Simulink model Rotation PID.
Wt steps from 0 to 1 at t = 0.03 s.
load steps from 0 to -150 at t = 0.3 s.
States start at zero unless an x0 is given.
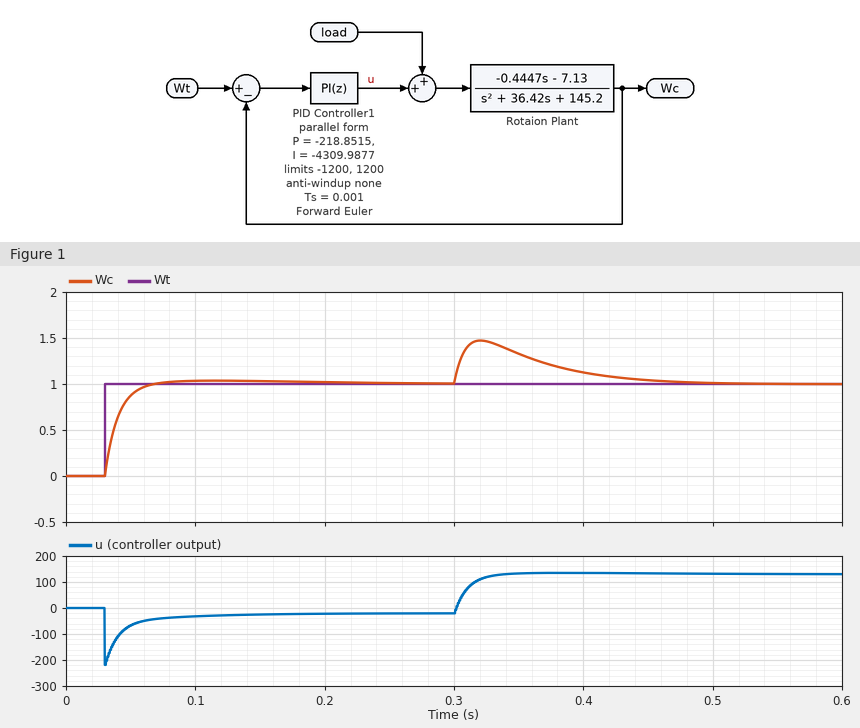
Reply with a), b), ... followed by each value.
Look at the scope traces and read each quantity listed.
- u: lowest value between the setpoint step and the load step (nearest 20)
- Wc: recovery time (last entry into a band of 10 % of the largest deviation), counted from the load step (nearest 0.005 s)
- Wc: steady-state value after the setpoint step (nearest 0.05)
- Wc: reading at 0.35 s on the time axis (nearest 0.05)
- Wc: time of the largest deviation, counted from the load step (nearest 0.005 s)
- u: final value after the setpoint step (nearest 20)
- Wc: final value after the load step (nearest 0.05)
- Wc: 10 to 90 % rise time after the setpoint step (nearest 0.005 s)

a) -220
b) 0.145 s
c) 1.00
d) 1.35
e) 0.020 s
f) -20
g) 1.00
h) 0.020 s
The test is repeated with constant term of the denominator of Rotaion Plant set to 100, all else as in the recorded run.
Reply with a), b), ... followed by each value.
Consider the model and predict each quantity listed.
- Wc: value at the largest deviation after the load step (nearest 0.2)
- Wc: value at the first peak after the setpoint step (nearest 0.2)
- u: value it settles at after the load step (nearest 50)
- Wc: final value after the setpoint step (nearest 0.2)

a) 1.4
b) 1.0
c) 150
d) 1.0
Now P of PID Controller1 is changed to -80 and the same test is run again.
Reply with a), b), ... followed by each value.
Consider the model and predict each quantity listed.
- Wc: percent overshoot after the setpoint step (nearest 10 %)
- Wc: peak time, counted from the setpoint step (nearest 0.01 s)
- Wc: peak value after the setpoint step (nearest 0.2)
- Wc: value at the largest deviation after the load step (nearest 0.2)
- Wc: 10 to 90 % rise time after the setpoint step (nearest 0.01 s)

a) 20 %
b) 0.07 s
c) 1.2
d) 1.8
e) 0.03 s
